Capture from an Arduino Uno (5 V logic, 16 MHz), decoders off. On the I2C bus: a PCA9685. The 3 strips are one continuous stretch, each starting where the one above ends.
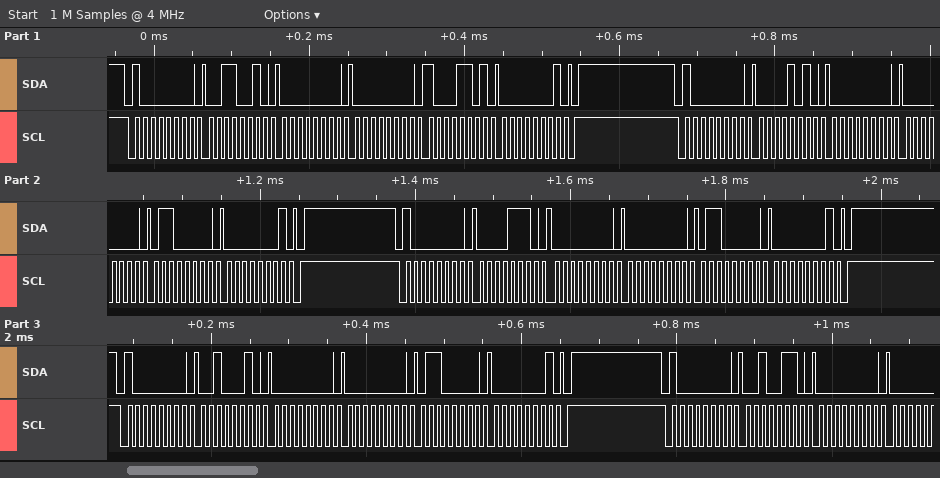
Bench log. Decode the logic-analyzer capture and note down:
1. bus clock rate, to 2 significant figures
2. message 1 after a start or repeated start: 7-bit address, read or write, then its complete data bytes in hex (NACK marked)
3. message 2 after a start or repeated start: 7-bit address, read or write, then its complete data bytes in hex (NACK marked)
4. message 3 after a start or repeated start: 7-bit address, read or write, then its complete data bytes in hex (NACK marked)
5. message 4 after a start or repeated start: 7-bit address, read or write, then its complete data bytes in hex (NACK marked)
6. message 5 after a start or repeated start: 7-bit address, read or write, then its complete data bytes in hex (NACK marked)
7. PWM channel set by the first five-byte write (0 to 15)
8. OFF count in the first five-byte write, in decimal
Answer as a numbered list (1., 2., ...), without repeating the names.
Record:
1. 100 kHz
2. 0x40 write: 32 00 00 8D 01
3. 0x40 write: 0A 00 00 60 01
4. 0x40 write: 0E 00 00 60 01
5. 0x40 write: 22 00 00 60 01
6. 0x40 write: 26 00
7. 11
8. 397
